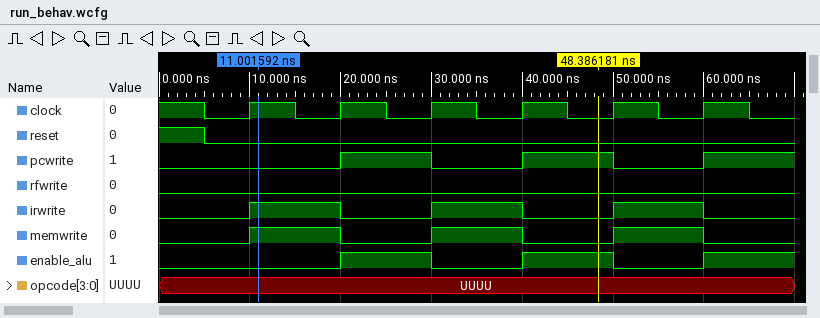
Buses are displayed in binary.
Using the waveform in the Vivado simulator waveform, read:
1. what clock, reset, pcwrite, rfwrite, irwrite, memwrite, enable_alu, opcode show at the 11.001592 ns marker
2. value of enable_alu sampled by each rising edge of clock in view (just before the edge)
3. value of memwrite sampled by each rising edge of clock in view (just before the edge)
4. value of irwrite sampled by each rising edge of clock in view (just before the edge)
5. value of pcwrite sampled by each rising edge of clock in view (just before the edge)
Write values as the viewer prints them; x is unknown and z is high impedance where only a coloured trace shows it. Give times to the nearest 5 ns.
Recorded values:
clock=1, reset=0, pcwrite=0, rfwrite=0, irwrite=1, memwrite=1, enable_alu=0, opcode=UUUU
0 0 1 0 1 0
0 1 0 1 0 1
0 1 0 1 0 1
0 0 1 0 1 0
